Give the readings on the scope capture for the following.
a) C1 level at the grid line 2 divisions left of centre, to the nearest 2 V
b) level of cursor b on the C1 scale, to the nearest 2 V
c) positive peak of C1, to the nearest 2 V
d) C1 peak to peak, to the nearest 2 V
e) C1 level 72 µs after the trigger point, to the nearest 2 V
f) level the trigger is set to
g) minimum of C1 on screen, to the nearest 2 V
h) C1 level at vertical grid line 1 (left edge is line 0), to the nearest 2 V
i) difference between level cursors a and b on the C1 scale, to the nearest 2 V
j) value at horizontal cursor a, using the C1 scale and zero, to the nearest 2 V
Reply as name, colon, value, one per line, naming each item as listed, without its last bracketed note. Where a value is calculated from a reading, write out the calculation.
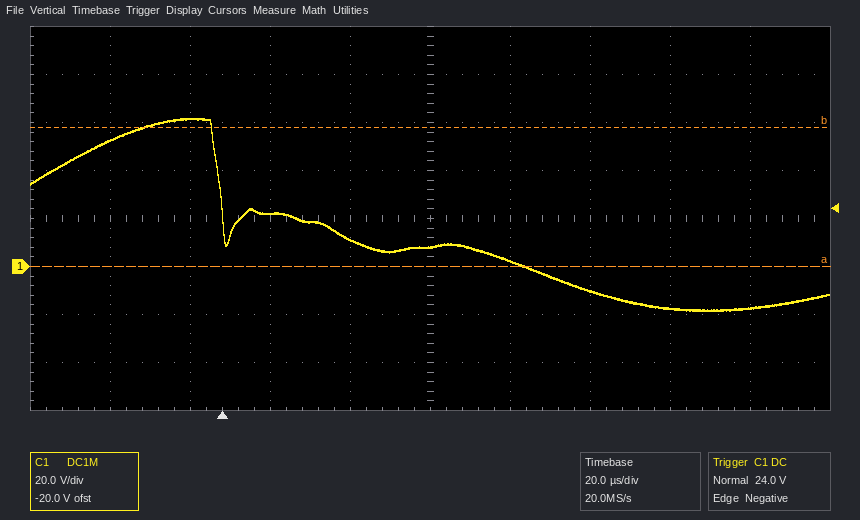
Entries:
C1 level at the grid line 2 divisions left of centre, to the nearest 2 V: 22 V
level of cursor b on the C1 scale, to the nearest 2 V: 58 V
positive peak of C1, to the nearest 2 V: 62 V
C1 peak to peak, to the nearest 2 V: 62 V − (-18 V) = 80 V
C1 level 72 µs after the trigger point, to the nearest 2 V: 2 V
level the trigger is set to: 24.0 V
minimum of C1 on screen, to the nearest 2 V: -18 V
C1 level at vertical grid line 1 (left edge is line 0), to the nearest 2 V: 52 V
difference between level cursors a and b on the C1 scale, to the nearest 2 V: 58 V
value at horizontal cursor a, using the C1 scale and zero, to the nearest 2 V: 0 V
